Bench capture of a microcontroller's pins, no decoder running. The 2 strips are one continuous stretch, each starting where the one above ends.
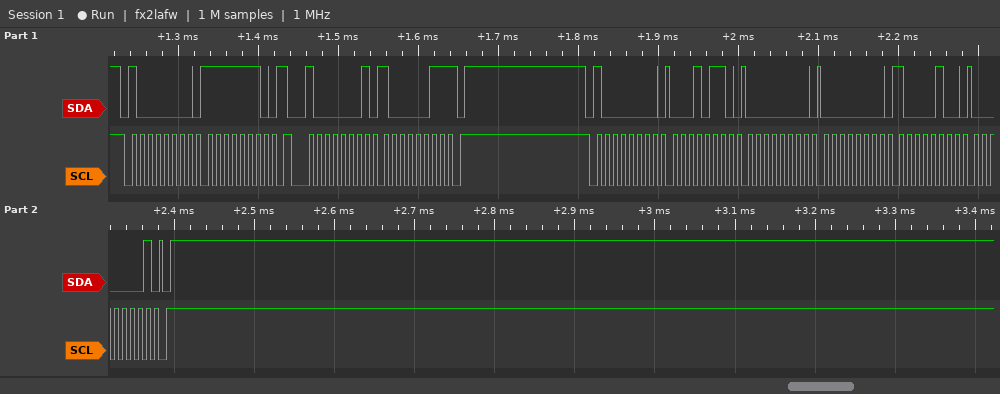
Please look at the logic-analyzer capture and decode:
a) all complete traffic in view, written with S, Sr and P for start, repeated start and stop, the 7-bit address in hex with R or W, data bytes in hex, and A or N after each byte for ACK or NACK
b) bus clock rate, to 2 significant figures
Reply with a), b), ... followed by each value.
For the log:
a) S 40W A FE A Sr 40R A 83 N P S 40W A 16 A 00 A 00 A 84 A 01 A P
b) 100 kHz
